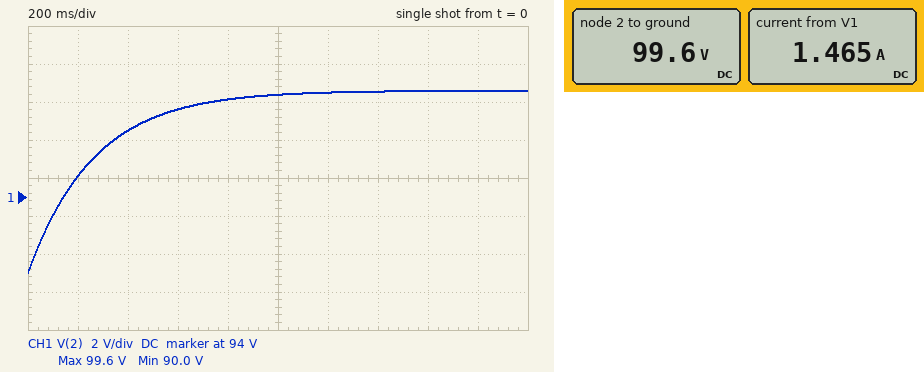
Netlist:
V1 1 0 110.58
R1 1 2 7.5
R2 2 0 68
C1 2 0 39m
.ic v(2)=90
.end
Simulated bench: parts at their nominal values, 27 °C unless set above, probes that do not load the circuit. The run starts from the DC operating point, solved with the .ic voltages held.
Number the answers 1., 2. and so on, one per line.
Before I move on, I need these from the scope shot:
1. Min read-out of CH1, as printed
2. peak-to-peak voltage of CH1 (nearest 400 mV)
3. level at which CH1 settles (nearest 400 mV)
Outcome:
1. 90.0 V
2. 9.6 V
3. 99.6 V
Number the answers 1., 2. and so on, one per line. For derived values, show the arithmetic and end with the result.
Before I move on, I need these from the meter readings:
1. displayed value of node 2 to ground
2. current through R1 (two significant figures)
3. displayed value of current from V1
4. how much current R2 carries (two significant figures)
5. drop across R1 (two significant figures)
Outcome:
1. 99.6 V
2. (110.6 V - 99.6 V) / 7.5 Ω = 1.5 A
3. 1.465 A
4. (99.6 V) / 68 Ω = 1.5 A
5. 110.6 V - 99.6 V = 11 V
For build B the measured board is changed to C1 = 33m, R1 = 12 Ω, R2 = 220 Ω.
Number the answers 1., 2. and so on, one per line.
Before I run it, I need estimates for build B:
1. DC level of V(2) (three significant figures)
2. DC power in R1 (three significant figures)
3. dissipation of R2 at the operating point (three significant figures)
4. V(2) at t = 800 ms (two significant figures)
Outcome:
1. 105 V
2. 2.73 W
3. 50.0 W
4. 100 V
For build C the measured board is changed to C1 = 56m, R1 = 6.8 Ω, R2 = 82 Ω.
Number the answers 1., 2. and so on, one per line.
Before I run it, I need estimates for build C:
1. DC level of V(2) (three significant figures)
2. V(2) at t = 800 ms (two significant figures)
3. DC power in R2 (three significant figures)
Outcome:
1. 102 V
2. 100 V
3. 127 W
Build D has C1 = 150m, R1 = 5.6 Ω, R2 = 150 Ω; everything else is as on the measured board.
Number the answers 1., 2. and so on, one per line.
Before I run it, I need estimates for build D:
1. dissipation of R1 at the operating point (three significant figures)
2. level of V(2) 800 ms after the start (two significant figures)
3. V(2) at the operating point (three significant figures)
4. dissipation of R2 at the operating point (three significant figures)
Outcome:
1. 2.83 W
2. 100 V
3. 107 V
4. 75.8 W
